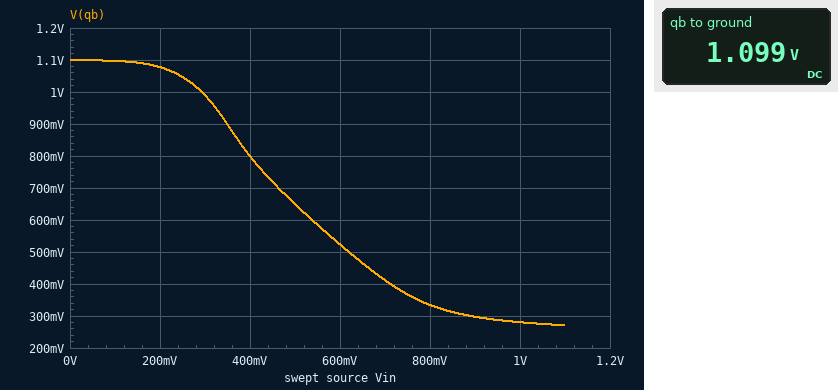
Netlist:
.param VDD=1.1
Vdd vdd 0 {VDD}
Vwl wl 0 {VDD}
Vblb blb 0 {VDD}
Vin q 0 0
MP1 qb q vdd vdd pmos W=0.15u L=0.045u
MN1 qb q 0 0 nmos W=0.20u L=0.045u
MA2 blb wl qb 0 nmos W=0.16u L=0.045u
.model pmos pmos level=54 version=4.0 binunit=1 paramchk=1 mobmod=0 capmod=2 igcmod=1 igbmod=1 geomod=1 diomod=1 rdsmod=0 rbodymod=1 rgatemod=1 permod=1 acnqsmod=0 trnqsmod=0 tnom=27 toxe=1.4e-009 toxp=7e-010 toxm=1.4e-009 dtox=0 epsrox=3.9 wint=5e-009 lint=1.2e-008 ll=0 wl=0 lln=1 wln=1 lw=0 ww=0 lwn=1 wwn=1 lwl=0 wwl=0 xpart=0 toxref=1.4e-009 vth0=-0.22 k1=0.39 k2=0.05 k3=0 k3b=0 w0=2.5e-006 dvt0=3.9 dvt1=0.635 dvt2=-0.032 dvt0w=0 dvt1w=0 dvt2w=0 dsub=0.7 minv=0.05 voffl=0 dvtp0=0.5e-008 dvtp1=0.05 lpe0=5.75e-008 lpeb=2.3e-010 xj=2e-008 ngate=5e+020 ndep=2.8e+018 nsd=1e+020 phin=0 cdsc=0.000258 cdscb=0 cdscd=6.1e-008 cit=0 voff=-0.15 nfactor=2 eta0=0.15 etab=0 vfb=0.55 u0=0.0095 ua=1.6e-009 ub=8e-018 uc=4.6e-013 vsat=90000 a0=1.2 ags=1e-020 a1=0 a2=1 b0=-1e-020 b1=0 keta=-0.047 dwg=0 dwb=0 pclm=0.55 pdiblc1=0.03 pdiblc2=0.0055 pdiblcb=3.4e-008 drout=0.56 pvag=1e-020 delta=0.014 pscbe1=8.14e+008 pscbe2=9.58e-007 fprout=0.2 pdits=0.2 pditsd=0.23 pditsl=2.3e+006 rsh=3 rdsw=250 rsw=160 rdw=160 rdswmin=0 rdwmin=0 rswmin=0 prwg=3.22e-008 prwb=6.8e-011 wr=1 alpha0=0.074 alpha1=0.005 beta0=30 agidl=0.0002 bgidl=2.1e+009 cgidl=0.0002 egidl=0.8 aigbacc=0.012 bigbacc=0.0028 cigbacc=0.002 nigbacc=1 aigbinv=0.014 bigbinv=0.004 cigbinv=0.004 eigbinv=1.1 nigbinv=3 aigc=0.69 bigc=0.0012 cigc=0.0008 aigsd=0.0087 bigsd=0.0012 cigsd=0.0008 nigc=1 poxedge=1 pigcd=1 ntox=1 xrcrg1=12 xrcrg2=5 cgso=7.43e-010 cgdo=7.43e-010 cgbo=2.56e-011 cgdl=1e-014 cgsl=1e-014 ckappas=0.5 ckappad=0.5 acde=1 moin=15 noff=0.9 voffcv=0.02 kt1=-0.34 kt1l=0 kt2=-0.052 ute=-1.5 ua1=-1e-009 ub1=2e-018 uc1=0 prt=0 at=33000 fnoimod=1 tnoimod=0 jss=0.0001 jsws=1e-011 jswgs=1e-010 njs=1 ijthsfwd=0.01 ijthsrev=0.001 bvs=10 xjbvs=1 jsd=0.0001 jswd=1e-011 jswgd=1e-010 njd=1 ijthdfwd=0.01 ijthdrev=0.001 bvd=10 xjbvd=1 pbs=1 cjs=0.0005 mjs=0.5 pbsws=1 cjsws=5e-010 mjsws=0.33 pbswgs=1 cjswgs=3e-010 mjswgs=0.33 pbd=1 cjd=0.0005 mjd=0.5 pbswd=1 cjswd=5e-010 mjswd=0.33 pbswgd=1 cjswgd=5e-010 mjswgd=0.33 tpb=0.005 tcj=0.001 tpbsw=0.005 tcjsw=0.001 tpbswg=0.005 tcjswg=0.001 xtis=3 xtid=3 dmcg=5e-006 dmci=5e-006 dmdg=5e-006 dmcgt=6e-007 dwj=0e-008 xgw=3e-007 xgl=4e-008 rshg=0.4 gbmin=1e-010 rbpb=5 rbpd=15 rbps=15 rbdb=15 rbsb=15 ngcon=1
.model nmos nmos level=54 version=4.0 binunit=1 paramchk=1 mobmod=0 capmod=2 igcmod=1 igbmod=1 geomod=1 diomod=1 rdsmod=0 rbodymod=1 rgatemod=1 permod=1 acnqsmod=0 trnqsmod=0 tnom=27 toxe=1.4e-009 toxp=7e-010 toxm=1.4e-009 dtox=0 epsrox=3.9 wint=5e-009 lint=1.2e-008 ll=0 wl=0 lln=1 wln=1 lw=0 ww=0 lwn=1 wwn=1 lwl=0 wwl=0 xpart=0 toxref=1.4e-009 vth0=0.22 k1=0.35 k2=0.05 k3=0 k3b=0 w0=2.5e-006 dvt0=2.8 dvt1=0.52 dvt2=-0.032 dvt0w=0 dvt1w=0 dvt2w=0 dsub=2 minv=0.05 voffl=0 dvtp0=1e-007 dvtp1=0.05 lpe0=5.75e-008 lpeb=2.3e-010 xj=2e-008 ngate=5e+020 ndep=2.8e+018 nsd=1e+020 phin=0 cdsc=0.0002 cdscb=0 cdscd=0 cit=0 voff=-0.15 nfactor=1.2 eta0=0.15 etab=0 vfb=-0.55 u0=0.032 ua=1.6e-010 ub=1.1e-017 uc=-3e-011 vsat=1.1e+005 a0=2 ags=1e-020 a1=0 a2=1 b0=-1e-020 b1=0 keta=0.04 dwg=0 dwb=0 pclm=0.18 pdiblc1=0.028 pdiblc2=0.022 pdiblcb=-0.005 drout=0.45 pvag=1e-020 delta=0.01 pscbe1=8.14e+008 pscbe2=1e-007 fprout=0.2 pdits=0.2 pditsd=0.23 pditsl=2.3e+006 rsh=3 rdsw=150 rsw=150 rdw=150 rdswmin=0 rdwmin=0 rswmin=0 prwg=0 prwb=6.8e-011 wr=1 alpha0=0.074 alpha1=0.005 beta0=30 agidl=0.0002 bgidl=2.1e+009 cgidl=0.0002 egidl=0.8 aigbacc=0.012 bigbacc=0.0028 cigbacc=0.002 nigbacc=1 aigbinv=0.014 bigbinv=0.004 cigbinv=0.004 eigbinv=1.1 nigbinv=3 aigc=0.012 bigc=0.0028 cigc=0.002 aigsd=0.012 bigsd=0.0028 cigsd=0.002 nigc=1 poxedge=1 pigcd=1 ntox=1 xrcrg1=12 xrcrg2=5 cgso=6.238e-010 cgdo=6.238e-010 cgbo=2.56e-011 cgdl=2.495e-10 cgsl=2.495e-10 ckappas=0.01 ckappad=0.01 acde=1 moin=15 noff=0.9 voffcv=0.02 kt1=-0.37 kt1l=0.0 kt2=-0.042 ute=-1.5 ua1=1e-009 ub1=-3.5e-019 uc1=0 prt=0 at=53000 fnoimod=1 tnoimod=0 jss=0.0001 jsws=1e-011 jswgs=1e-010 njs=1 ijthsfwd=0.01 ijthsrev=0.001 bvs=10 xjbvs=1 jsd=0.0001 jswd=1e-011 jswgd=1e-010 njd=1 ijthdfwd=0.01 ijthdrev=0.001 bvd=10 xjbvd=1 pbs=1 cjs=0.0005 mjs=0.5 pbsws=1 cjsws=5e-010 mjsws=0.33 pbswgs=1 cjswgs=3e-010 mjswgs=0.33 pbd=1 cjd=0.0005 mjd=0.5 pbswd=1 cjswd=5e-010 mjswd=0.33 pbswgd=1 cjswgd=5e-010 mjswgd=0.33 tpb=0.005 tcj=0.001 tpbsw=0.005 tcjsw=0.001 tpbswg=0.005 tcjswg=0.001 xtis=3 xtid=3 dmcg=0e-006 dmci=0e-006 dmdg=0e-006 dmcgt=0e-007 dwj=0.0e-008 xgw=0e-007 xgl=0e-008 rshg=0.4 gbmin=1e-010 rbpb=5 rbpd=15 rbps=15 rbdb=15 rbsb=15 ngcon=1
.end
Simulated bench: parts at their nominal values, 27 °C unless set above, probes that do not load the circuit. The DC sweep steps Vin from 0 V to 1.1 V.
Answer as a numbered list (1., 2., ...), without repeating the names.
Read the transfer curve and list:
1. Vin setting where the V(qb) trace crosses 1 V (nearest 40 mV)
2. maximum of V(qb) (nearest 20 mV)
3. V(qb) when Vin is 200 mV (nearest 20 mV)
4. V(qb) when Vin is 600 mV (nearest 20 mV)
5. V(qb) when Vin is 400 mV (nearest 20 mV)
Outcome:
1. 280 mV
2. 1.10 V
3. 1.08 V
4. 520 mV
5. 800 mV
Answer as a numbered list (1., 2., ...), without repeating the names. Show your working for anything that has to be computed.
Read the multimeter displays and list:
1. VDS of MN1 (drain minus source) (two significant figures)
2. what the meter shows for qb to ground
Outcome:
1. 1.099 V = 1.1 V
2. 1.099 V
